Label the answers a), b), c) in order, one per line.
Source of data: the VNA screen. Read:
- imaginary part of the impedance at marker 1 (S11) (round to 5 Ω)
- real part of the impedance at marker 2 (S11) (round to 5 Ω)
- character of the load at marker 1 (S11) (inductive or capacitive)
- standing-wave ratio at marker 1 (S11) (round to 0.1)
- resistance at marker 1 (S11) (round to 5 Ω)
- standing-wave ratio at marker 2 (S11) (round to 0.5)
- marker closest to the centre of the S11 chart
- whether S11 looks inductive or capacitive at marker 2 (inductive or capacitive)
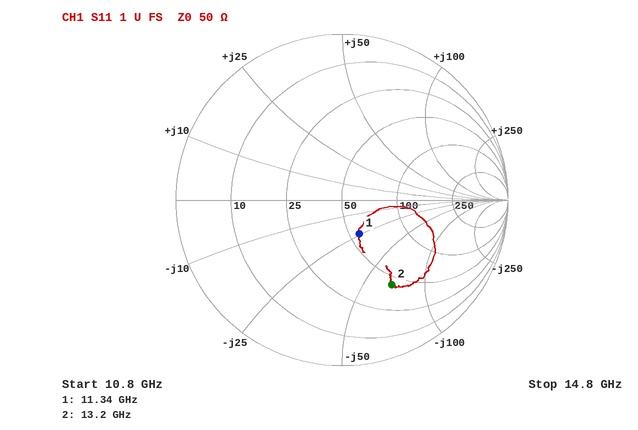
a) -25 Ω
b) 45 Ω
c) capacitive
d) 1.6
e) 55 Ω
f) 4.0
g) marker 1
h) capacitive
